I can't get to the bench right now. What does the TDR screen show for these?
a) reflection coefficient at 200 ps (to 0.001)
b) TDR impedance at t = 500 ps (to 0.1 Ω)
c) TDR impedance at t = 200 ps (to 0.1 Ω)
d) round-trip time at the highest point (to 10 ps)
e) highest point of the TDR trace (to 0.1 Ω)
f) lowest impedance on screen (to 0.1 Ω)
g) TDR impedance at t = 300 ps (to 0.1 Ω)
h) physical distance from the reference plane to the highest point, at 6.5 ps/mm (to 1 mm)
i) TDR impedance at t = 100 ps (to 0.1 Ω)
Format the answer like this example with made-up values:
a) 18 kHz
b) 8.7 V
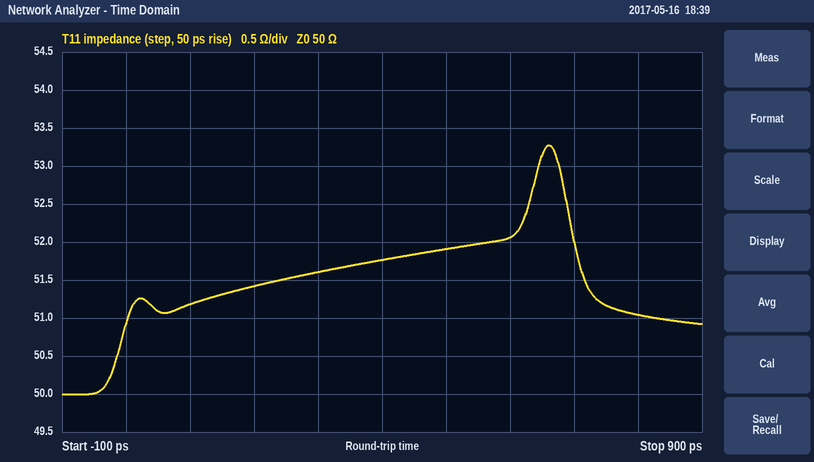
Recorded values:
a) +0.014
b) 51.9 Ω
c) 51.4 Ω
d) 660 ps
e) 53.3 Ω
f) 50.0 Ω
g) 51.6 Ω
h) 51 mm
i) 51.2 Ω
